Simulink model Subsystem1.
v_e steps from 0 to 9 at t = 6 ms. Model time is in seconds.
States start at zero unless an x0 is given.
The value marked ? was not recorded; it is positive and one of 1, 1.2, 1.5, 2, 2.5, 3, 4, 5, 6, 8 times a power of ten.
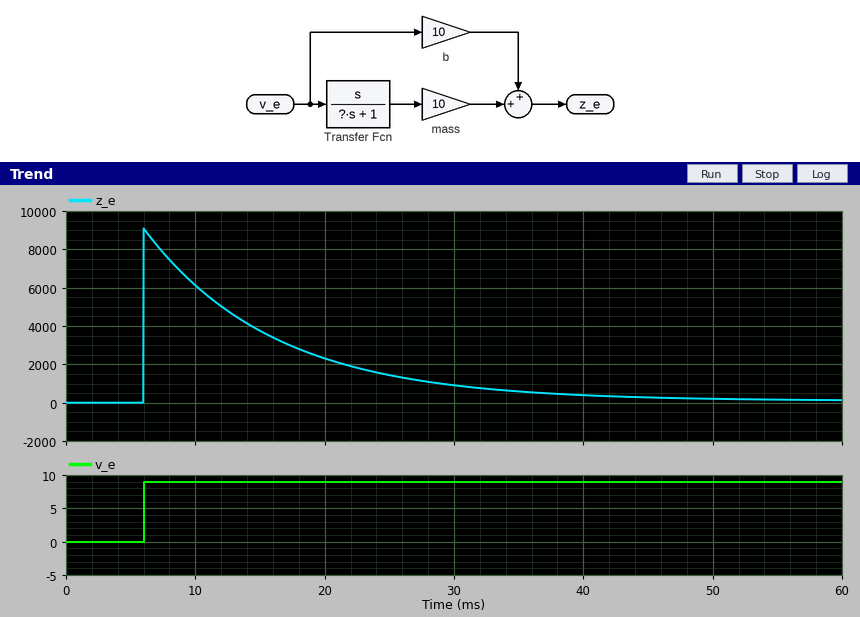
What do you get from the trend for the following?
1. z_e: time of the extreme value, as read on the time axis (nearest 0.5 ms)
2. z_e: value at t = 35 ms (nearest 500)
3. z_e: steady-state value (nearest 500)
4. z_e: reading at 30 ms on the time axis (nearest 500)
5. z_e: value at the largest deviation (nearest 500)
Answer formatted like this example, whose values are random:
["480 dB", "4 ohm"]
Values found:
["6.0 ms", "500", "0", "1000", "9000"]
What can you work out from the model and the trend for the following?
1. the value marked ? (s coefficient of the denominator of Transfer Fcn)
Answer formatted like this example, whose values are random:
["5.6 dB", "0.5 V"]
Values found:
["0.01"]
